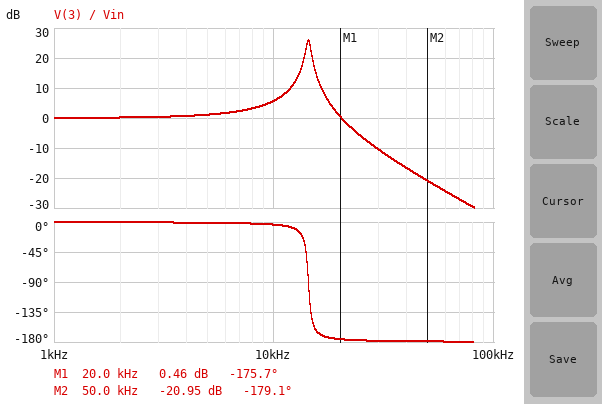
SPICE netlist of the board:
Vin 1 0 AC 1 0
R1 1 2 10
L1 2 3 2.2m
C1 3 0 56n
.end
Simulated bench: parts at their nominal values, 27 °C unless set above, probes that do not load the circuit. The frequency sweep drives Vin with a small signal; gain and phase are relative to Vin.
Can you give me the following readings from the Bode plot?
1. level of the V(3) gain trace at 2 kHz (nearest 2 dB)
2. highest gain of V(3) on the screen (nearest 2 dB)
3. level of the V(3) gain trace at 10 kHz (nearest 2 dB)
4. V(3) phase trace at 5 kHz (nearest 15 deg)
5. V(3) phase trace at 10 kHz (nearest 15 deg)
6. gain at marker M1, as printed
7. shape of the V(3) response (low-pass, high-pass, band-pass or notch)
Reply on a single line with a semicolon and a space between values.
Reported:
0 dB; 26 dB; 6 dB; 0 deg; 0 deg; 0.46 dB; low-pass
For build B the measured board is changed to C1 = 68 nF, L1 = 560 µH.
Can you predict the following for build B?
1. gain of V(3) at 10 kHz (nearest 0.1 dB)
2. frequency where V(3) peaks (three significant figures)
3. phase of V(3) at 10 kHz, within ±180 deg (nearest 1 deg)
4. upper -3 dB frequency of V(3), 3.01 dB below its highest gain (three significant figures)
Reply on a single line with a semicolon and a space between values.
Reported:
1.4 dB; 25.7 kHz; -3 deg; 27.1 kHz
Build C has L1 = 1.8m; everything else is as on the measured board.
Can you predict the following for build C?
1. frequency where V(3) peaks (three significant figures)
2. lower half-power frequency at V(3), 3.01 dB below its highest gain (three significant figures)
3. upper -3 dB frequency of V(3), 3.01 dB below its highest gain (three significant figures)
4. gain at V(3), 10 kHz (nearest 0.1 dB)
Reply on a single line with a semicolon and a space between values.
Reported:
15.8 kHz; 15.4 kHz; 16.3 kHz; 4.4 dB
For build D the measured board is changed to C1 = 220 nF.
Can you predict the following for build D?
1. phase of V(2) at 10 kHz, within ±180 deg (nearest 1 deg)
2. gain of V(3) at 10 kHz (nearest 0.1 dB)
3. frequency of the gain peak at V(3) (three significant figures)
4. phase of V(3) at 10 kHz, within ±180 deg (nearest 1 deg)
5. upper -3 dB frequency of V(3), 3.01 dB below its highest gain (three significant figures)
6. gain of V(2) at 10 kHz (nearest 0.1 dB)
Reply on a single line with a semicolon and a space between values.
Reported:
9 deg; 0.7 dB; 7.22 kHz; -171 deg; 7.57 kHz; -0.1 dB
